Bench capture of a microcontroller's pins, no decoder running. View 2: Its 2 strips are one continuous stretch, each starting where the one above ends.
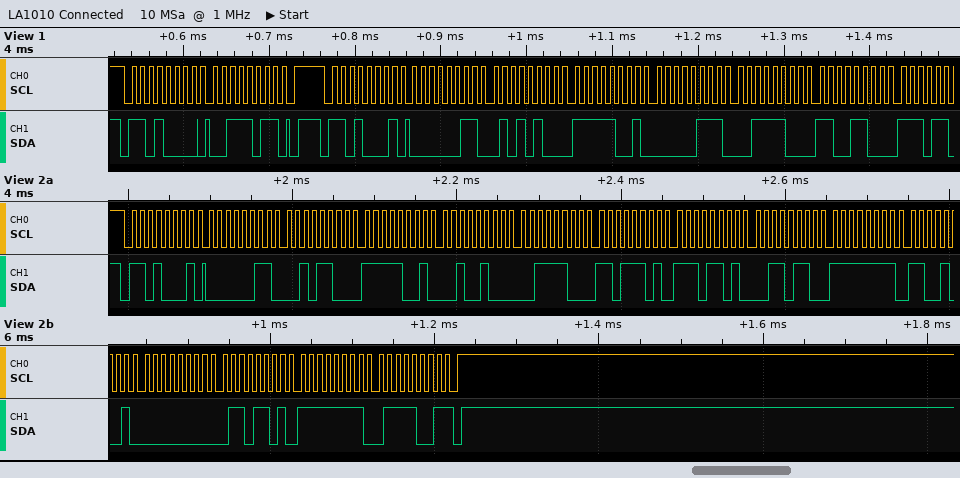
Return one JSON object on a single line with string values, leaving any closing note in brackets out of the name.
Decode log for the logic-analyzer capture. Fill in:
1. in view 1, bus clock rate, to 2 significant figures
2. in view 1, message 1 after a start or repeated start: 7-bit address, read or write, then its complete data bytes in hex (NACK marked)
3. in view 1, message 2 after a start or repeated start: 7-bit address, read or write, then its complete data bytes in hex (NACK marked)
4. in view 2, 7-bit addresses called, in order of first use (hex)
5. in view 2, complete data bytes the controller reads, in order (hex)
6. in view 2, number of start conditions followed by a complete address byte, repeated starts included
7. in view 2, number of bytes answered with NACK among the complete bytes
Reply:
{"in view 1, bus clock rate, to 2 significant figures": "100 kHz", "in view 1, message 1 after a start or repeated start: 7-bit address, read or write, then its complete data bytes in hex": "0x68 write: 3B", "in view 1, message 2 after a start or repeated start: 7-bit address, read or write, then its complete data bytes in hex": "0x68 read: 03 54 F9 07 3C CC", "in view 2, 7-bit addresses called, in order of first use": "0x68", "in view 2, complete data bytes the controller reads, in order": "03 2C F9 24 3C DD ED 36 FF C9 00 6D FF 79", "in view 2, number of start conditions followed by a complete address byte, repeated starts included": "1", "in view 2, number of bytes answered with NACK among the complete bytes": "1"}
